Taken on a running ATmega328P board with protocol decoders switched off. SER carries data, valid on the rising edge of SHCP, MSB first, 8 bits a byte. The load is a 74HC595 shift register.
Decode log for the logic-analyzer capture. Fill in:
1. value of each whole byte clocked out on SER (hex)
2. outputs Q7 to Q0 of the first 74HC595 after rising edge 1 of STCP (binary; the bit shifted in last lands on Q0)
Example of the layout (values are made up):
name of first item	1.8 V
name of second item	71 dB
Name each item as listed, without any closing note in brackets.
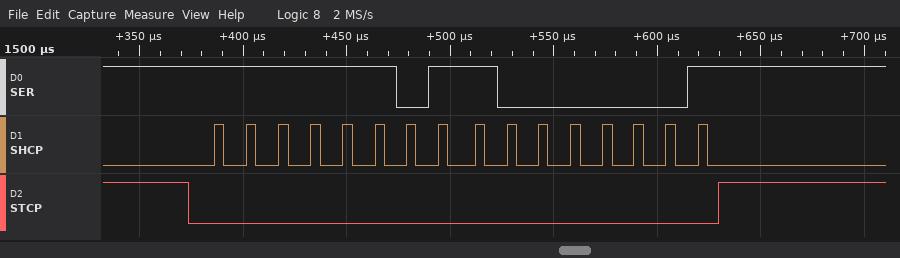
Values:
value of each whole byte clocked out on SER	0xFD 0x81
outputs Q7 to Q0 of the first 74HC595 after rising edge 1 of STCP	10000001
